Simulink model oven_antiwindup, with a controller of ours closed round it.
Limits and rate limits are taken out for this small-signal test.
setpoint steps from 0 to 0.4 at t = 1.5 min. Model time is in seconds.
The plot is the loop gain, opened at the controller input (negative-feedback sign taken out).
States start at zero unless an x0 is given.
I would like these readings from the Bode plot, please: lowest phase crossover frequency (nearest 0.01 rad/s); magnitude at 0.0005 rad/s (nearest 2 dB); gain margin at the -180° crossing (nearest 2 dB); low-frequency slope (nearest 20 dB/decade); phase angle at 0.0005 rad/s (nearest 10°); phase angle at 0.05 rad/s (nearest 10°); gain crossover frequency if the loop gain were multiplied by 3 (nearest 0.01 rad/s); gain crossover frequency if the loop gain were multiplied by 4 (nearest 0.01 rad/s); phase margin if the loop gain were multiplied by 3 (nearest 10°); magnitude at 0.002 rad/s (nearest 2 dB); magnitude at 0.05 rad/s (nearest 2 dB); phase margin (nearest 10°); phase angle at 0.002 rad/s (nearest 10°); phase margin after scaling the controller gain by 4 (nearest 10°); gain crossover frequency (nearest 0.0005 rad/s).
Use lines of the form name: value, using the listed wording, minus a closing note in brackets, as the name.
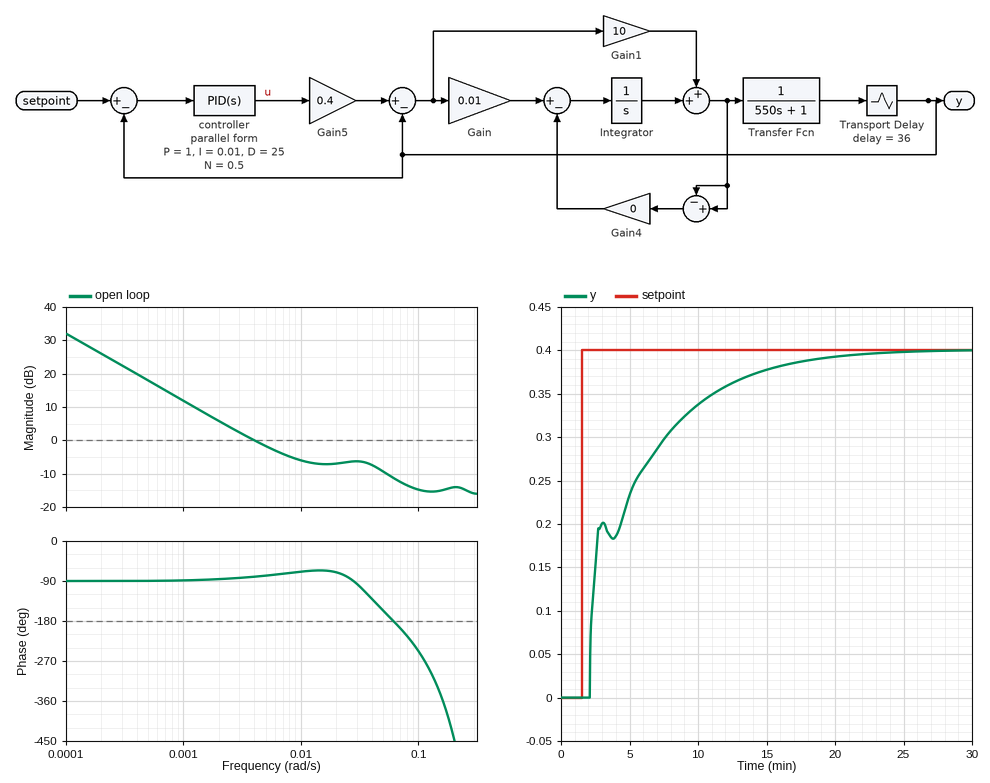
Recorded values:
lowest phase crossover frequency: 0.06 rad/s
magnitude at 0.0005 rad/s: 18 dB
gain margin at the -180° crossing: 12 dB
low-frequency slope: -20 dB/decade
phase angle at 0.0005 rad/s: -90°
phase angle at 0.05 rad/s: -160°
gain crossover frequency if the loop gain were multiplied by 3: 0.05 rad/s
gain crossover frequency if the loop gain were multiplied by 4: 0.07 rad/s
phase margin if the loop gain were multiplied by 3: 20°
magnitude at 0.002 rad/s: 6 dB
magnitude at 0.05 rad/s: -10 dB
phase margin: 100°
phase angle at 0.002 rad/s: -90°
phase margin after scaling the controller gain by 4: -10°
gain crossover frequency: 0.0040 rad/s
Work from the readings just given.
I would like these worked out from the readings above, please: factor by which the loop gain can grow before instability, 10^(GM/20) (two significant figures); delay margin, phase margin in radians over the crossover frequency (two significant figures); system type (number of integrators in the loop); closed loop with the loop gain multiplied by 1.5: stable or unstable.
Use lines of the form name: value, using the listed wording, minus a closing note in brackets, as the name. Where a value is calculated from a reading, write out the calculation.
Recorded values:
factor by which the loop gain can grow before instability, 10^(GM/20): 10^(12 / 20) = 4.0
delay margin, phase margin in radians over the crossover frequency: 100 × π / 180 / 0.004 = 440 s
system type: 1
closed loop with the loop gain multiplied by 1.5: stable or unstable: stable
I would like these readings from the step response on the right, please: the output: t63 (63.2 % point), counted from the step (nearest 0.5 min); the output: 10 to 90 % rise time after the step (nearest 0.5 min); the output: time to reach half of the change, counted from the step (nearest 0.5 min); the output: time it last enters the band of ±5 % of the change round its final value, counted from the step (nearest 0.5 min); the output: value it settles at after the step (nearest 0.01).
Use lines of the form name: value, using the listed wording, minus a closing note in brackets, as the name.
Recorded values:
the output: t63 (63.2 % point), counted from the step: 4.0 min
the output: 10 to 90 % rise time after the step: 10.0 min
the output: time to reach half of the change, counted from the step: 1.5 min
the output: time it last enters the band of ±5 % of the change round its final value, counted from the step: 14.0 min
the output: value it settles at after the step: 0.40
